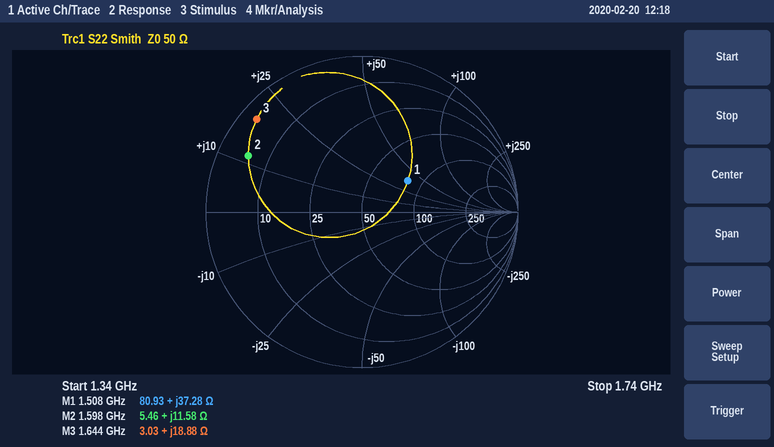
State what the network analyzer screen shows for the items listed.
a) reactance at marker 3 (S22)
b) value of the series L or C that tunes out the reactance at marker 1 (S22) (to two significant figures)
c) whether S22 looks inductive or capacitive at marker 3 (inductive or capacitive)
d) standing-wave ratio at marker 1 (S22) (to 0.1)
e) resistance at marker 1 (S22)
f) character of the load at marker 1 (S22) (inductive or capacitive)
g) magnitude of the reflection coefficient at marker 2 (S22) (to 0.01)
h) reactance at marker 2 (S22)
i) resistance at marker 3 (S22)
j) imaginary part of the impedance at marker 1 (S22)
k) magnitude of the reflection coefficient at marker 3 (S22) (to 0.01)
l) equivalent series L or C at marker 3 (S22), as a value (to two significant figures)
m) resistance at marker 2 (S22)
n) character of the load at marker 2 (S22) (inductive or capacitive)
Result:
+18.88 Ω
2.8 pF
inductive
2.1
80.93 Ω
inductive
0.81
+11.58 Ω
3.03 Ω
+37.28 Ω
0.90
1.8 nH
5.46 Ω
inductive
